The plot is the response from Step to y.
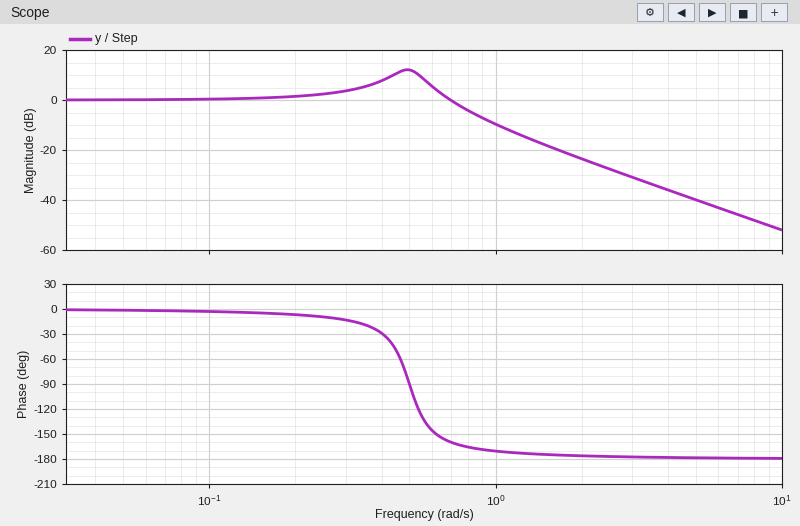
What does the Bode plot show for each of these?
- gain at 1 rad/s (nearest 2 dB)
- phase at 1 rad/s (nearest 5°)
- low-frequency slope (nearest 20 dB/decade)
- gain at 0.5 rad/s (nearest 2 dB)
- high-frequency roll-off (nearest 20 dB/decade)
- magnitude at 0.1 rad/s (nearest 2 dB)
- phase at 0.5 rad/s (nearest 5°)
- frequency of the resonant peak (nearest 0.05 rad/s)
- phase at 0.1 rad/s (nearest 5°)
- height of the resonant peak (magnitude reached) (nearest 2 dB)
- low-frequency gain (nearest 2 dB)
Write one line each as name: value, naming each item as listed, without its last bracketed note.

gain at 1 rad/s: -10 dB
phase at 1 rad/s: -170°
low-frequency slope: 0 dB/decade
gain at 0.5 rad/s: 12 dB
high-frequency roll-off: -40 dB/decade
magnitude at 0.1 rad/s: 0 dB
phase at 0.5 rad/s: -90°
frequency of the resonant peak: 0.50 rad/s
phase at 0.1 rad/s: -5°
height of the resonant peak (magnitude reached): 12 dB
low-frequency gain: 0 dB
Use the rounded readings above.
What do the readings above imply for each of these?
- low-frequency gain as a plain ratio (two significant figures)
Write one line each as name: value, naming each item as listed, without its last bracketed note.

low-frequency gain as a plain ratio: 1.0
